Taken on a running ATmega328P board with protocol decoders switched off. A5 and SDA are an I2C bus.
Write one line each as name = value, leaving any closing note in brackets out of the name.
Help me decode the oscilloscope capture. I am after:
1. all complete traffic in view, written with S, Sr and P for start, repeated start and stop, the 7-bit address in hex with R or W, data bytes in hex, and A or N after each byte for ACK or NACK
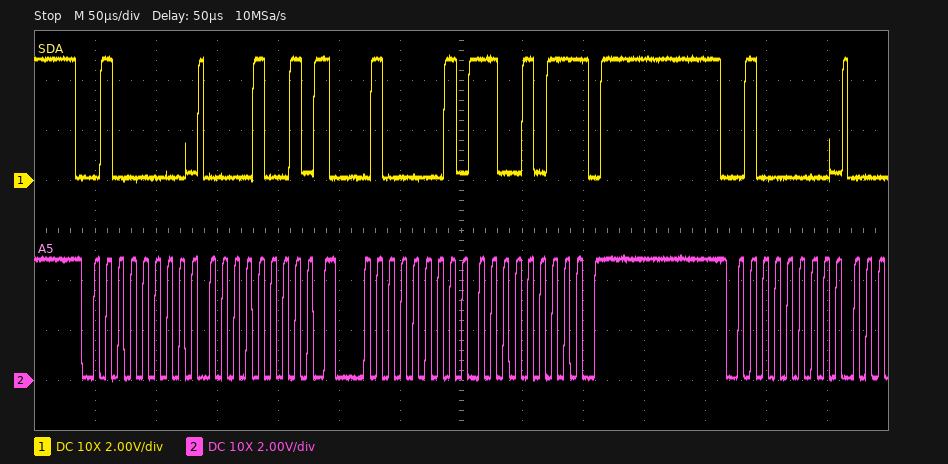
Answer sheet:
all complete traffic in view, written with S, Sr and P for start, repeated start and stop, the 7-bit address in hex with R or W, data bytes in hex, and A or N after each byte for ACK or NACK = S 20W A 09 A Sr 20R A CB N P S 20W A
